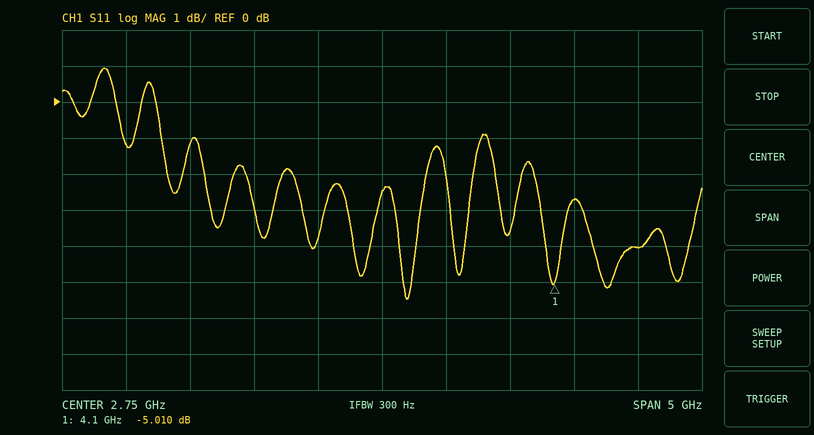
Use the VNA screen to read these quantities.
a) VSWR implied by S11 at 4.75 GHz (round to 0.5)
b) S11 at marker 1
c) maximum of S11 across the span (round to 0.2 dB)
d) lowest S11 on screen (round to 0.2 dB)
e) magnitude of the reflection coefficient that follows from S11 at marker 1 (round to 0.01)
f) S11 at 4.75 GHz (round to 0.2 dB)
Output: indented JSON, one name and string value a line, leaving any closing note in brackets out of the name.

{
  "VSWR implied by S11 at 4.75 GHz": "4.5",
  "S11 at marker 1": "-5.010 dB",
  "maximum of S11 across the span": "1.0 dB",
  "lowest S11 on screen": "-5.4 dB",
  "magnitude of the reflection coefficient that follows from S11 at marker 1": "0.56",
  "S11 at 4.75 GHz": "-4.0 dB"
}
